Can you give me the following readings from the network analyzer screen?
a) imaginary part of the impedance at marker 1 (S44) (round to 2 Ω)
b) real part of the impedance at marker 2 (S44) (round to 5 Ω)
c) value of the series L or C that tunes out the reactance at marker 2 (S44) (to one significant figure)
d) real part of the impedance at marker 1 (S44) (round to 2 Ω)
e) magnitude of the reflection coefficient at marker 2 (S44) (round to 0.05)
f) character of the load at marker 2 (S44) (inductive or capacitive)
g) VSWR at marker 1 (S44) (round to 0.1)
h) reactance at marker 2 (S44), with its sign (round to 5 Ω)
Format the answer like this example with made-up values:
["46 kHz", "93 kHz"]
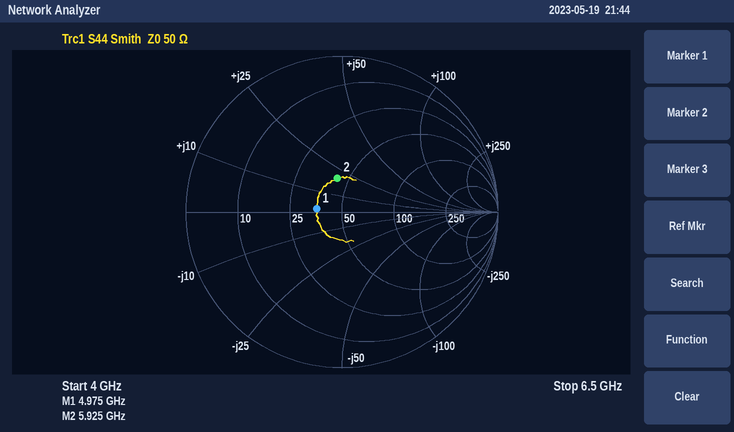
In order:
["+2 Ω", "45 Ω", "1 pF", "36 Ω", "0.20", "inductive", "1.4", "+20 Ω"]
